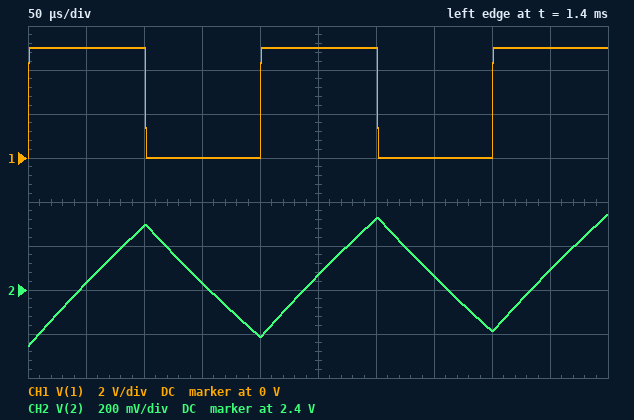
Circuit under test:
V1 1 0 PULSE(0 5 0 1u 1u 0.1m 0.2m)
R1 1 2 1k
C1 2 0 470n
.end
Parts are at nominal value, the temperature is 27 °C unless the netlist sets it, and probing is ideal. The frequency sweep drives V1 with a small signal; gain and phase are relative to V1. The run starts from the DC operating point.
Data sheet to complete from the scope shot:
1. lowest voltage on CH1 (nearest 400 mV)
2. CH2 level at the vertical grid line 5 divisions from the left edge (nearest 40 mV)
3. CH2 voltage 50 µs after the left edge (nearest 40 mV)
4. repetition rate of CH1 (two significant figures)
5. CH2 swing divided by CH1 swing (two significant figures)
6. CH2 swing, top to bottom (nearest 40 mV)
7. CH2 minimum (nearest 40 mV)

0 V
2.48 V
2.44 V
5.0 kHz
0.12
600 mV
2.16 V
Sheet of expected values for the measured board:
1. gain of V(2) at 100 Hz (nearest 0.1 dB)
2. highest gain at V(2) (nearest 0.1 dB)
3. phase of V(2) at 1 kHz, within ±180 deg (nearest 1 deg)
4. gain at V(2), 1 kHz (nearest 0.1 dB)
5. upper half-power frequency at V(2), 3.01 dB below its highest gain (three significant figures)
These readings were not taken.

-0.4 dB
0 dB
-71 deg
-9.9 dB
339 Hz
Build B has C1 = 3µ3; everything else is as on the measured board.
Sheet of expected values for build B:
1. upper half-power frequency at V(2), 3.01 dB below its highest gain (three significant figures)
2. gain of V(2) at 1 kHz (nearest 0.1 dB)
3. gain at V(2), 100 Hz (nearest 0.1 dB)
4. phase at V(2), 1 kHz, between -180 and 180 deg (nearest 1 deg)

48.2 Hz
-26.3 dB
-7.2 dB
-87 deg
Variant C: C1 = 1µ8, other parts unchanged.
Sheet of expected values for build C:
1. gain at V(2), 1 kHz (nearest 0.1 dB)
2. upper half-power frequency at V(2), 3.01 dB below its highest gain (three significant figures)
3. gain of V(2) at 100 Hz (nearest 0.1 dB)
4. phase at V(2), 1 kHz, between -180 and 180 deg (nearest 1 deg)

-21.1 dB
88.4 Hz
-3.6 dB
-85 deg
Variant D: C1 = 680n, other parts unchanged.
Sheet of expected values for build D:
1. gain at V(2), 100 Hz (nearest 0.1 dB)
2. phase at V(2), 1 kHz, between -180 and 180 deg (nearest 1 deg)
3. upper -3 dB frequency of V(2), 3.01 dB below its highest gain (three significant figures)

-0.7 dB
-77 deg
234 Hz
